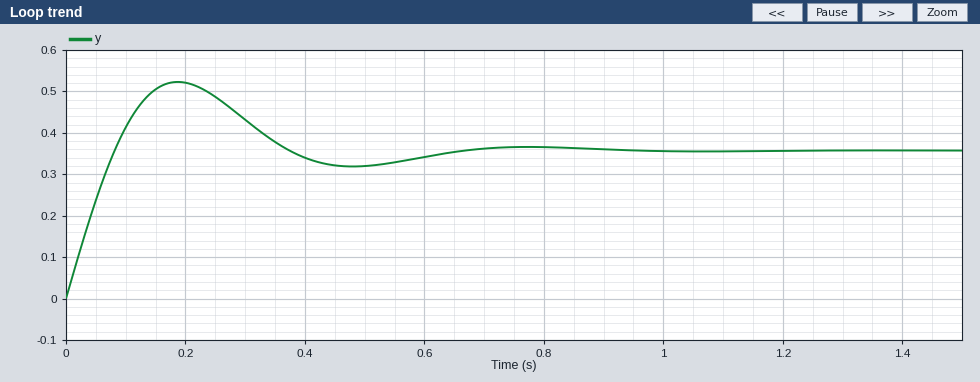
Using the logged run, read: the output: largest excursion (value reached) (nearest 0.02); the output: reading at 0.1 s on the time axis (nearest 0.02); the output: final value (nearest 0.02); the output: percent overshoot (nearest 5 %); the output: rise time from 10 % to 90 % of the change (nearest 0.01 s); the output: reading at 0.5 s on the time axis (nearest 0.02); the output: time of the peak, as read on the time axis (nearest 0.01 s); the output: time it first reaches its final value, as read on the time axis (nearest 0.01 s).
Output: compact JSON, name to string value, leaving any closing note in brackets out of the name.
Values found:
{"the output: largest excursion (value reached)": "0.52", "the output: reading at 0.1 s on the time axis": "0.42", "the output: final value": "0.36", "the output: percent overshoot": "45 %", "the output: rise time from 10 % to 90 % of the change": "0.06 s", "the output: reading at 0.5 s on the time axis": "0.32", "the output: time of the peak, as read on the time axis": "0.19 s", "the output: time it first reaches its final value, as read on the time axis": "0.08 s"}
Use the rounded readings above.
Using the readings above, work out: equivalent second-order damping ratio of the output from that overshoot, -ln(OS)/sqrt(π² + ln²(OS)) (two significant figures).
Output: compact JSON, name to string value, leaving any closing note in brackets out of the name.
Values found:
{"equivalent second-order damping ratio of the output from that overshoot, -ln(OS)/sqrt(π² + ln²(OS))": "0.25"}
